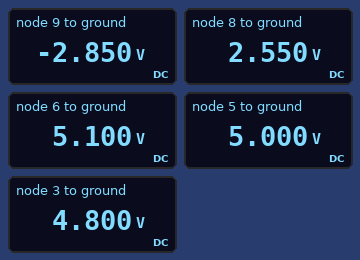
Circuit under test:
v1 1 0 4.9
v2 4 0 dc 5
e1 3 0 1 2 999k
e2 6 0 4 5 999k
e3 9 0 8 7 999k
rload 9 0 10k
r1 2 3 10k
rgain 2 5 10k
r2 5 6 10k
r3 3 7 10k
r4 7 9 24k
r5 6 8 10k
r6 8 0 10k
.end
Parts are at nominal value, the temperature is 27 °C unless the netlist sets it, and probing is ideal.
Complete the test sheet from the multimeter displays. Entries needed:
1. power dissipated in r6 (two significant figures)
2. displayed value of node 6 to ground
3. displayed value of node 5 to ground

650 µW
5.100 V
5.000 V
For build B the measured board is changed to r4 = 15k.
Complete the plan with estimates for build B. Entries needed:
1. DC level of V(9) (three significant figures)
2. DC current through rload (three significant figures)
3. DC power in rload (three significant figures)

-825 mV
82.5 µA
68.1 µW
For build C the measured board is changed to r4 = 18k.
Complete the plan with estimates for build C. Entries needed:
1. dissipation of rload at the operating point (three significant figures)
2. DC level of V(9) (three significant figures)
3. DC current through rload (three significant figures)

225 µW
-1.50 V
150 µA
